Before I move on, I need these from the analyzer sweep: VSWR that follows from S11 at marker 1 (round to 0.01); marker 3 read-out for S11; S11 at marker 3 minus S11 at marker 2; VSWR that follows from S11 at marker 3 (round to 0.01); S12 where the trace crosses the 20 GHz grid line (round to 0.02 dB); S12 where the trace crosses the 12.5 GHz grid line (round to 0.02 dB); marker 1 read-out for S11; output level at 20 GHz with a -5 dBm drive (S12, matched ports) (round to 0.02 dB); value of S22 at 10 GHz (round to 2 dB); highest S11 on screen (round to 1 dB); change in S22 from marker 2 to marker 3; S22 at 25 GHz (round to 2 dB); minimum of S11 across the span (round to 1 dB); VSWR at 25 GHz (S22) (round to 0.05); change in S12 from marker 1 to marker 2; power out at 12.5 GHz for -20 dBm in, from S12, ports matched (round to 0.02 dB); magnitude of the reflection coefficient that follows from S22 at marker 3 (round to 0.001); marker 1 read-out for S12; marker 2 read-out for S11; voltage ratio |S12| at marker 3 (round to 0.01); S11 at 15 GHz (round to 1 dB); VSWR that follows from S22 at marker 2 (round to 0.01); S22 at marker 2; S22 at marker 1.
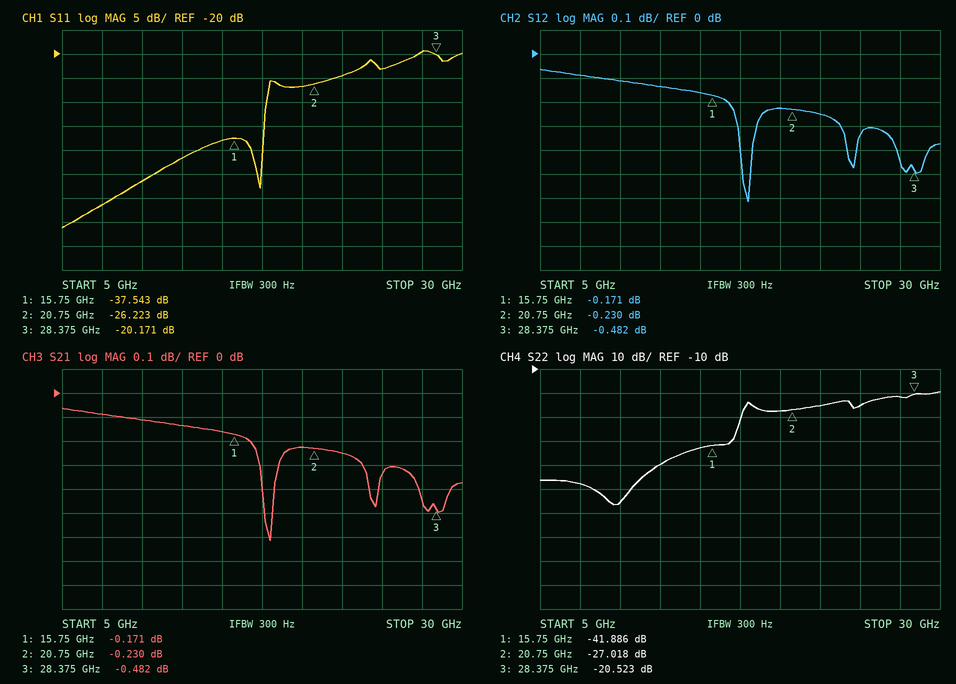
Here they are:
1.03
-20.171 dB
6.052 dB
1.22
-0.22 dB
-0.14 dB
-37.543 dB
-5.22 dBm
-66 dB
-19 dB
6.495 dB
-26 dB
-56 dB
1.10
-0.059 dB
-20.14 dBm
0.094
-0.171 dB
-26.223 dB
0.95
-38 dB
1.09
-27.018 dB
-41.886 dB
